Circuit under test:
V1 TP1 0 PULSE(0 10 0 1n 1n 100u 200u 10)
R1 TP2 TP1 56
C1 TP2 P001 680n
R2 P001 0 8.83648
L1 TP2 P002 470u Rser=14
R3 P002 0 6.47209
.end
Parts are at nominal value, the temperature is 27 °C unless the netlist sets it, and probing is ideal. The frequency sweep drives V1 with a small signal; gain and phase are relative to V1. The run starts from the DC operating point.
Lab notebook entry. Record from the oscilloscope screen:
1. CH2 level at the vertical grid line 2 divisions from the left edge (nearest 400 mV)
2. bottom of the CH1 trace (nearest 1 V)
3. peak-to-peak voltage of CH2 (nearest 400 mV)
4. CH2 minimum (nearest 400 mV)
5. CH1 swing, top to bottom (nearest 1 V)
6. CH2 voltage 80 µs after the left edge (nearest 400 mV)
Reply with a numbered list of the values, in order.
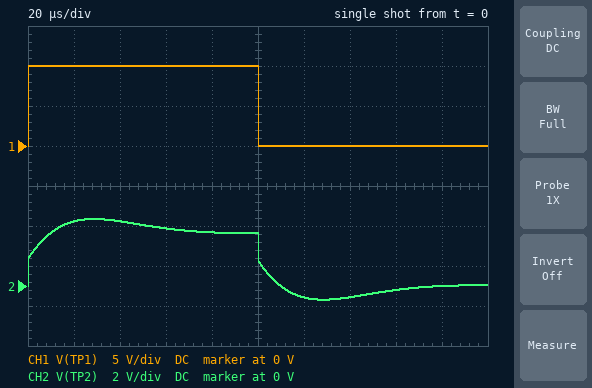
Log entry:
1. 3.2 V
2. 0 V
3. 4.0 V
4. -800 mV
5. 10 V
6. 2.8 V
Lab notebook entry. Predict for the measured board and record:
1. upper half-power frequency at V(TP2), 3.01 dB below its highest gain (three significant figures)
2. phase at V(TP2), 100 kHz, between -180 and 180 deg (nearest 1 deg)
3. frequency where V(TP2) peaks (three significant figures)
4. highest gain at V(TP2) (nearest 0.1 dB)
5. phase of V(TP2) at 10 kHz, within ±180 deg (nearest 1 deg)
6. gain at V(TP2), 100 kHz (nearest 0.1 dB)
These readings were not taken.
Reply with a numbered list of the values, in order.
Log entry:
1. 17.6 kHz
2. -11 deg
3. 8.29 kHz
4. -8.7 dB
5. -17 deg
6. -17.0 dB
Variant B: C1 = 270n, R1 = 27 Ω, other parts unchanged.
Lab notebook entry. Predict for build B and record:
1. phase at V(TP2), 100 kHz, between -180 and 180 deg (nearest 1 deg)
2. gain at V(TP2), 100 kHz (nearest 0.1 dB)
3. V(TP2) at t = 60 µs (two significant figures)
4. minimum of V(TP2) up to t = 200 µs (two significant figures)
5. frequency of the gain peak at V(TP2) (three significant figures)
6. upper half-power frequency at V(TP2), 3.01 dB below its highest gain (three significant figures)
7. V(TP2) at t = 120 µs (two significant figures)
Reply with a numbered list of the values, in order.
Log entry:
1. -23 deg
2. -10.6 dB
3. 4.3 V
4. -2.0 V
5. 15.0 kHz
6. 34.4 kHz
7. -1.7 V
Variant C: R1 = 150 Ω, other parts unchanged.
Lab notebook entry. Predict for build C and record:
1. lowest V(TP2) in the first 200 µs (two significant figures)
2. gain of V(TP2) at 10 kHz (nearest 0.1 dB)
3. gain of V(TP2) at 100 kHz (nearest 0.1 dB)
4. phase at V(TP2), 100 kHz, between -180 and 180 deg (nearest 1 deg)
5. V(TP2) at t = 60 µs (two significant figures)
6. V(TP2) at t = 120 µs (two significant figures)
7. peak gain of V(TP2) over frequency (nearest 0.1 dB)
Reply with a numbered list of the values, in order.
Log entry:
1. -370 mV
2. -15.4 dB
3. -24.8 dB
4. -12 deg
5. 1.3 V
6. -290 mV
7. -15.1 dB
